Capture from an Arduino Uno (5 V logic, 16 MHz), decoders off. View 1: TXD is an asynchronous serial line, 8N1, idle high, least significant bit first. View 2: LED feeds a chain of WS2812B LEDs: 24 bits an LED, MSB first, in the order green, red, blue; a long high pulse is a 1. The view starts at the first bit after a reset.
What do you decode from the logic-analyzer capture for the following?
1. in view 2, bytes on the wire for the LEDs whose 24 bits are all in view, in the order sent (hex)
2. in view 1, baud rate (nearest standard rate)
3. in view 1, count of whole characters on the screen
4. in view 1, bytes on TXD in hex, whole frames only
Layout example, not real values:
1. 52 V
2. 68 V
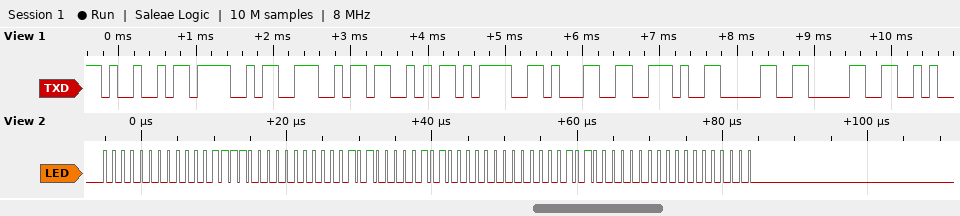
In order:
1. 00 0F 00 14 14 00 14 00 00
2. 9600 baud
3. 9
4. 0x49 0x4F 0x4E 0x53 0x3D 0x31 0x2E 0x30 0x30
